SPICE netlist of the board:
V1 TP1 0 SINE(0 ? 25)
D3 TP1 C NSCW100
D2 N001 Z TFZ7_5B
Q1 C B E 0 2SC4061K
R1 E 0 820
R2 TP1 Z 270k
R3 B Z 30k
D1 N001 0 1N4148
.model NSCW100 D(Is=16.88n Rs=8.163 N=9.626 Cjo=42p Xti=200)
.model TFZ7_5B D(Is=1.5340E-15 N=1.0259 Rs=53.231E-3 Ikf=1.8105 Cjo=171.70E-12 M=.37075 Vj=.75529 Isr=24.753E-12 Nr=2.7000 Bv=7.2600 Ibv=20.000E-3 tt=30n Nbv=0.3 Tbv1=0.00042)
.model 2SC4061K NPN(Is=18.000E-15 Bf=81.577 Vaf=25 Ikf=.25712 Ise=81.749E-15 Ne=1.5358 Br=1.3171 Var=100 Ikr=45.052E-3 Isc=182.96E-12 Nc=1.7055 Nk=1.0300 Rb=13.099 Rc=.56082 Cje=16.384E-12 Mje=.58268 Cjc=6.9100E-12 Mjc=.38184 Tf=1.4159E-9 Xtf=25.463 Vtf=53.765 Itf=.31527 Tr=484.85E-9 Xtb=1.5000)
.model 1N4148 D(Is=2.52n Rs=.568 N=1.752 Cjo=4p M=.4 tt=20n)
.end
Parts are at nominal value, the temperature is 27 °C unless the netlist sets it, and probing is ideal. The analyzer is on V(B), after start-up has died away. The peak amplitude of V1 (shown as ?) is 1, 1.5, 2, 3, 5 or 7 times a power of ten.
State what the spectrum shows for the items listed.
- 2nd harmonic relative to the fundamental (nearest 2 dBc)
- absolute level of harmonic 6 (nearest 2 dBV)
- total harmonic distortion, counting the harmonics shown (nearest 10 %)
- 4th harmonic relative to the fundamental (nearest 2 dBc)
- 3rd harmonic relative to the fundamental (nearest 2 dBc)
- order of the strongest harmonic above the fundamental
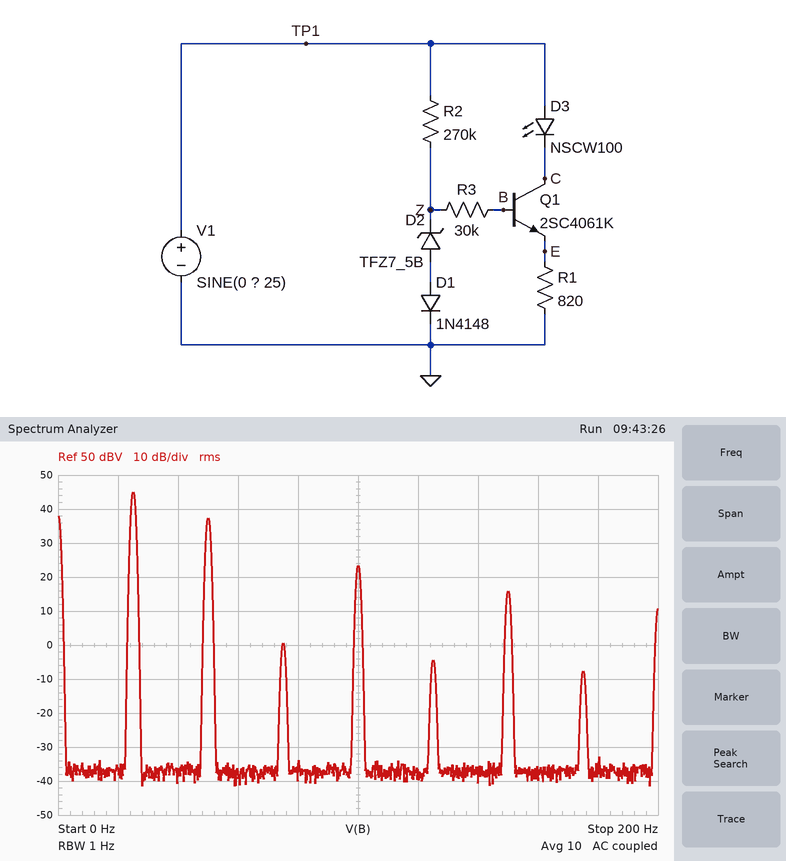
-8 dBc
16 dBV
40 %
-22 dBc
-44 dBc
2
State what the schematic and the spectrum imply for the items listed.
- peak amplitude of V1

500 V
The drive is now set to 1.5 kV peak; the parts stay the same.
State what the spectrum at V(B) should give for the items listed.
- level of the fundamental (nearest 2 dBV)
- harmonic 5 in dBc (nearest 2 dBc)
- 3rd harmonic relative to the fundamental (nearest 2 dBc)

54 dBV
-58 dBc
-54 dBc
